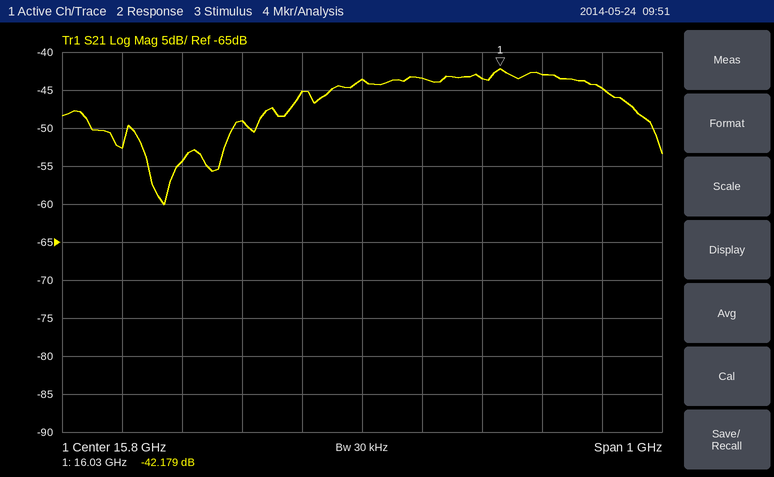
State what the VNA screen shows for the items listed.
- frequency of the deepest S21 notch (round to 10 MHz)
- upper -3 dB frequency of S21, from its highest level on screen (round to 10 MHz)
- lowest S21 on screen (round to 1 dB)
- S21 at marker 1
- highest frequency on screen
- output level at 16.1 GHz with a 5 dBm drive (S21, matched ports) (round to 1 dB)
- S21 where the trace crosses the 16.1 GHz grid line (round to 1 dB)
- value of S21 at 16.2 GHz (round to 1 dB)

15.47 GHz
16.21 GHz
-60 dB
-42.179 dB
16.3 GHz
-38 dBm
-43 dB
-45 dB
